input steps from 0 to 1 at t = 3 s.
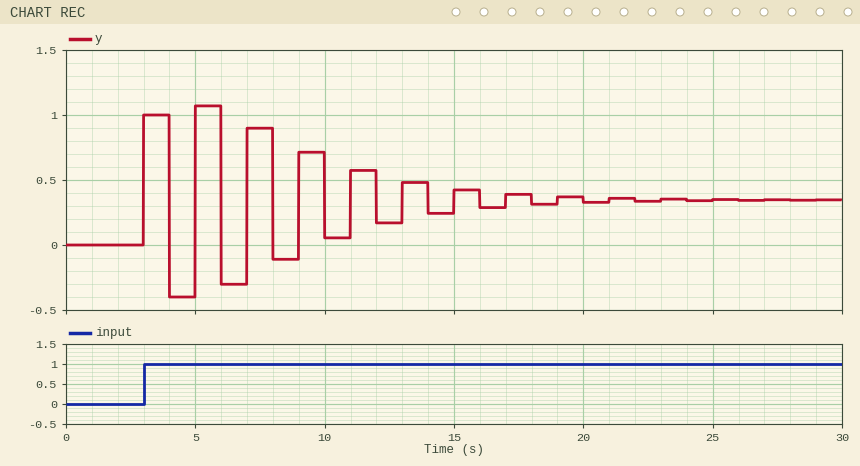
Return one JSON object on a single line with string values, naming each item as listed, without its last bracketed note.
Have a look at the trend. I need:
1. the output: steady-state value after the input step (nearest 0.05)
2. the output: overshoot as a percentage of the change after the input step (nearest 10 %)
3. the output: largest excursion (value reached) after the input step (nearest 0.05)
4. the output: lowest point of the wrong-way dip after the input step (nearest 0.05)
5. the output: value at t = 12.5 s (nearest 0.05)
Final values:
{"the output: steady-state value after the input step": "0.35", "the output: overshoot as a percentage of the change after the input step": "210 %", "the output: largest excursion (value reached) after the input step": "1.05", "the output: lowest point of the wrong-way dip after the input step": "-0.40", "the output: value at t = 12.5 s": "0.15"}
